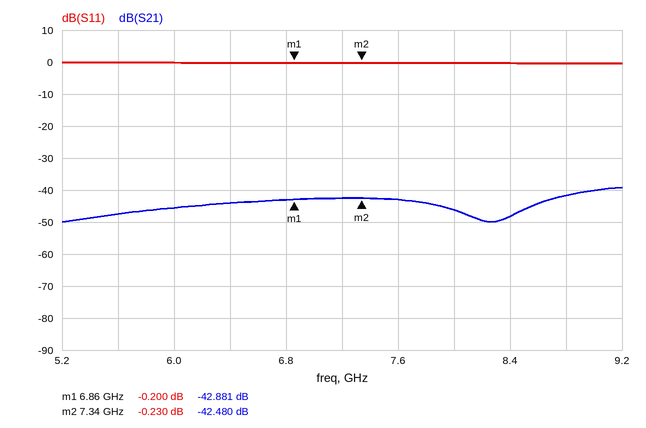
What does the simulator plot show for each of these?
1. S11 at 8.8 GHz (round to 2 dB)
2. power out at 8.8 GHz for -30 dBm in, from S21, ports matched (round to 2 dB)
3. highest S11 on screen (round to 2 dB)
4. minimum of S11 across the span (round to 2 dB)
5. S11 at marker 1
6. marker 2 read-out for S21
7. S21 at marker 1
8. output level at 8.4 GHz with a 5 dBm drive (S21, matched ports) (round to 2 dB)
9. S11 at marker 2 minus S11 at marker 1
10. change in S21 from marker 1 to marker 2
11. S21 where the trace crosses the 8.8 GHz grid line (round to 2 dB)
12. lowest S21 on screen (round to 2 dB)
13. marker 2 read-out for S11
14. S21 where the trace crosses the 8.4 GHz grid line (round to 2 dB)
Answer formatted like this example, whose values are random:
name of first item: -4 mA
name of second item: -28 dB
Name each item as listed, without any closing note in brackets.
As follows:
S11 at 8.8 GHz: 0 dB
power out at 8.8 GHz for -30 dBm in, from S21, ports matched: -72 dBm
highest S11 on screen: 0 dB
minimum of S11 across the span: 0 dB
S11 at marker 1: -0.200 dB
marker 2 read-out for S21: -42.480 dB
S21 at marker 1: -42.881 dB
output level at 8.4 GHz with a 5 dBm drive (S21, matched ports): -44 dBm
S11 at marker 2 minus S11 at marker 1: -0.030 dB
change in S21 from marker 1 to marker 2: 0.401 dB
S21 where the trace crosses the 8.8 GHz grid line: -42 dB
lowest S21 on screen: -50 dB
marker 2 read-out for S11: -0.230 dB
S21 where the trace crosses the 8.4 GHz grid line: -48 dB
